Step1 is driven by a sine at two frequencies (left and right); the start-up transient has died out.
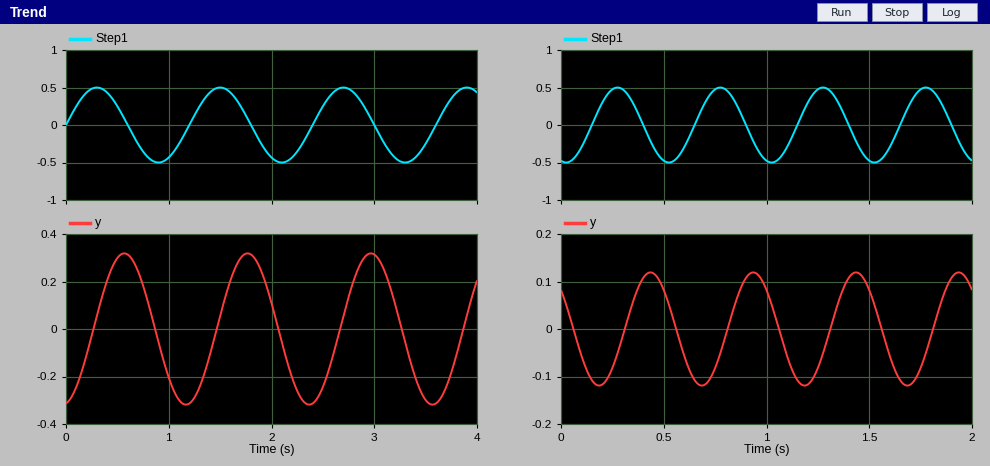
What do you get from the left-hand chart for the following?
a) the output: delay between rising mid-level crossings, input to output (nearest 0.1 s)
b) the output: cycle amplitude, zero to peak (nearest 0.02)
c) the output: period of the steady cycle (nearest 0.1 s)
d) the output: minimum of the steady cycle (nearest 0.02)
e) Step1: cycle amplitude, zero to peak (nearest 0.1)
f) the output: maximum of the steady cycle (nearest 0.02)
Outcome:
0.3 s
0.32
1.2 s
-0.32
0.5
0.32
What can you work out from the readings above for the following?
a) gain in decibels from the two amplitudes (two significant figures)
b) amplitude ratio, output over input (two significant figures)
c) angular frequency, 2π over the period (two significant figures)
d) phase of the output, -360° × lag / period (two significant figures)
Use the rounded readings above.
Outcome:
-3.9 dB
0.64
5.2 rad/s
-90°
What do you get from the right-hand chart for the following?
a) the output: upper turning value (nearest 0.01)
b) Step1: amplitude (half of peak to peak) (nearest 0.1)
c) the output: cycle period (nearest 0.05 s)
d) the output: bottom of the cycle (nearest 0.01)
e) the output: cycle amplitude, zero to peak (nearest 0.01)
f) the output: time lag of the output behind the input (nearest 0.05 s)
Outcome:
0.12
0.5
0.50 s
-0.12
0.12
0.15 s
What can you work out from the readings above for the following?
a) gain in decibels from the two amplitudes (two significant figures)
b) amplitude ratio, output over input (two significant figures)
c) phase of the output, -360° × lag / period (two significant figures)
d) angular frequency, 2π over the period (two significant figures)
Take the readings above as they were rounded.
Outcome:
-12 dB
0.24
-110°
13 rad/s
